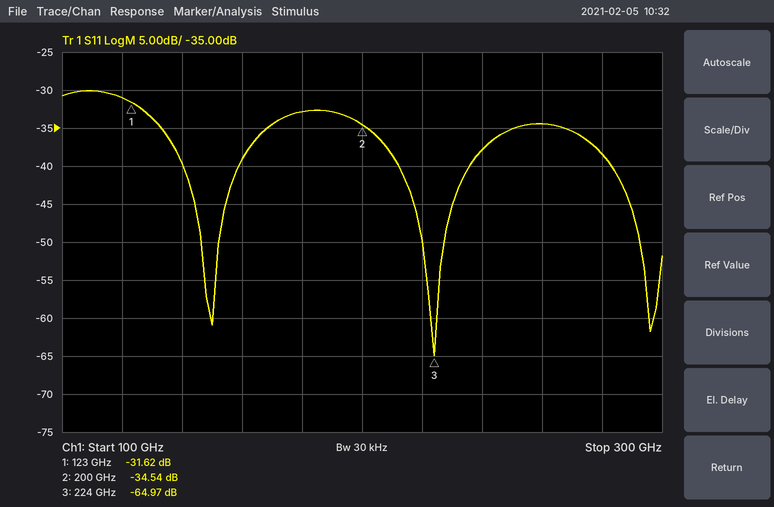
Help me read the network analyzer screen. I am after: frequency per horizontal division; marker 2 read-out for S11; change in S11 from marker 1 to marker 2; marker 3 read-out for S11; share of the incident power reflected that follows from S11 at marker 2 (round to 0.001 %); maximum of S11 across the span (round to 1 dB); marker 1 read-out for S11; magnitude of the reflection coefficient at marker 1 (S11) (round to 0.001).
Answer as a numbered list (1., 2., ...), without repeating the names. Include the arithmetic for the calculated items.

1. 20 GHz
2. -34.54 dB
3. -34.54 − (-31.62) = -2.92 dB
4. -64.97 dB
5. 10^(-34.54/10) ≈ 0.035 %
6. -30 dB
7. -31.62 dB
8. 10^(-31.62/20) ≈ 0.026
